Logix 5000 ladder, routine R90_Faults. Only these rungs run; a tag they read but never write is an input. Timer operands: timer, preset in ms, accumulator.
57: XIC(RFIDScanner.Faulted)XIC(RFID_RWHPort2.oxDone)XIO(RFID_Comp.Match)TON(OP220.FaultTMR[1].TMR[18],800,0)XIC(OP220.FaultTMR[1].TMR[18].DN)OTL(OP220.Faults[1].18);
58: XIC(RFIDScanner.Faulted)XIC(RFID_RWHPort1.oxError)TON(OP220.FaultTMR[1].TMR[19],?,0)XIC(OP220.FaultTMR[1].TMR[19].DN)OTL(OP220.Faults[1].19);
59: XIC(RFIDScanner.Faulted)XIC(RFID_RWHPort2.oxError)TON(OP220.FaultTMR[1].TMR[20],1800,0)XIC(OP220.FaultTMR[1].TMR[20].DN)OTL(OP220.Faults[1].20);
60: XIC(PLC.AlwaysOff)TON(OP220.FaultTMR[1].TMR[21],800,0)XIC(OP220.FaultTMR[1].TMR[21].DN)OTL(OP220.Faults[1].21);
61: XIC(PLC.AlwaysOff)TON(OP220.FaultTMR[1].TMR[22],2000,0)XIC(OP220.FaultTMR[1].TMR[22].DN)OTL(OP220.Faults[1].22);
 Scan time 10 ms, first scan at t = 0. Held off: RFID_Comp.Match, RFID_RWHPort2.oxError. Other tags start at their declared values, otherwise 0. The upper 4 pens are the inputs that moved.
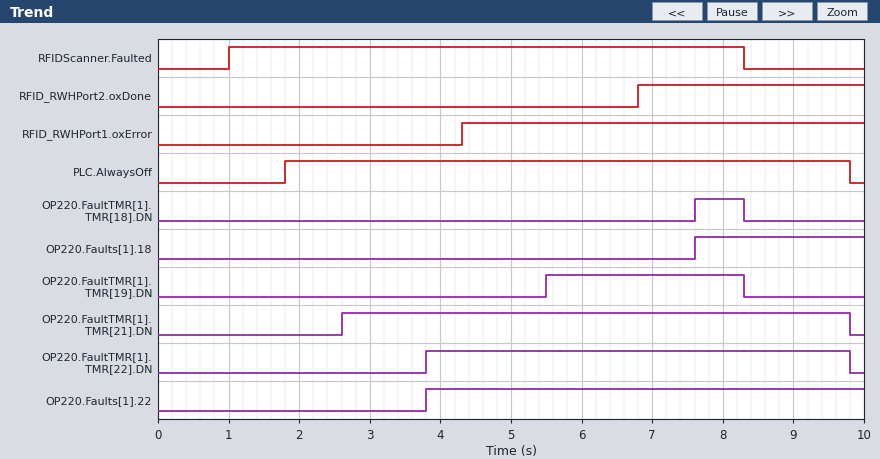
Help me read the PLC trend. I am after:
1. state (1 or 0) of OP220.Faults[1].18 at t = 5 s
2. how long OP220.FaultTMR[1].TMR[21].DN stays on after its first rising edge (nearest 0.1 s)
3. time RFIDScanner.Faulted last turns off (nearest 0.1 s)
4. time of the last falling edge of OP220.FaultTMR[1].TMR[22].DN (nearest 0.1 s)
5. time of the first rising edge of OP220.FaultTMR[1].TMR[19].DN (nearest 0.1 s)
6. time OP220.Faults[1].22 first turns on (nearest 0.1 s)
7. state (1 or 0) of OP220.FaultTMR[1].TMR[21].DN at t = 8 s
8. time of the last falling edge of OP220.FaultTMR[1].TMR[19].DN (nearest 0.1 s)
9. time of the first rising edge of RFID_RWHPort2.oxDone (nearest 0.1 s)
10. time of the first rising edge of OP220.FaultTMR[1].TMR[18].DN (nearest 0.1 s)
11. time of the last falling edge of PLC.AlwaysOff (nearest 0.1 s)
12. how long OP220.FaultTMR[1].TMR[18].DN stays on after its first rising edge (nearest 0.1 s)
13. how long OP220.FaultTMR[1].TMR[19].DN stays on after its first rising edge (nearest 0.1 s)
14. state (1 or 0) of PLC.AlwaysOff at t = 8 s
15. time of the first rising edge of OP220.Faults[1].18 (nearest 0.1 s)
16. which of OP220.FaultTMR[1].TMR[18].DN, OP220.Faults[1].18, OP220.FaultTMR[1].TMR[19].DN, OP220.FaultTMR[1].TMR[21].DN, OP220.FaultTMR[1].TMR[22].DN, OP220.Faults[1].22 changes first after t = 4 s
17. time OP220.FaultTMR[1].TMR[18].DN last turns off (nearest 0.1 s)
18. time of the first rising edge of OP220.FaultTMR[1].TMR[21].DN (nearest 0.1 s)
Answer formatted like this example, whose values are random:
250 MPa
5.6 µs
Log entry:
0
7.2 s
8.3 s
9.8 s
5.5 s
3.8 s
1
8.3 s
6.8 s
7.6 s
9.8 s
0.7 s
2.8 s
1
7.6 s
OP220.FaultTMR[1].TMR[19].DN
8.3 s
2.6 s
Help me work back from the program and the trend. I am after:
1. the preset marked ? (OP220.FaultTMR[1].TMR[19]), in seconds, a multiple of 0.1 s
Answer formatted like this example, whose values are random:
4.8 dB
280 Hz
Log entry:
1.2 s
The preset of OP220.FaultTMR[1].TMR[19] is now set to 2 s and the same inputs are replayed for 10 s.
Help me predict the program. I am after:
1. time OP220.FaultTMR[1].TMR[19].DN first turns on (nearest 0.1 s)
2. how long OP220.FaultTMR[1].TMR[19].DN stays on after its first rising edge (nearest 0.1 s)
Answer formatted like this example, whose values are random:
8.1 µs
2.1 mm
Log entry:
6.3 s
2.0 s
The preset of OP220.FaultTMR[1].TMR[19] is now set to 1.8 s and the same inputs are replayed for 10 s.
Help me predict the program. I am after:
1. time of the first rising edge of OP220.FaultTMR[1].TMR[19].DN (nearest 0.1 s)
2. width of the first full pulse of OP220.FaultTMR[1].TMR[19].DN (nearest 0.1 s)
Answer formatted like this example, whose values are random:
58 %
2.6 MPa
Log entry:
6.1 s
2.2 s
